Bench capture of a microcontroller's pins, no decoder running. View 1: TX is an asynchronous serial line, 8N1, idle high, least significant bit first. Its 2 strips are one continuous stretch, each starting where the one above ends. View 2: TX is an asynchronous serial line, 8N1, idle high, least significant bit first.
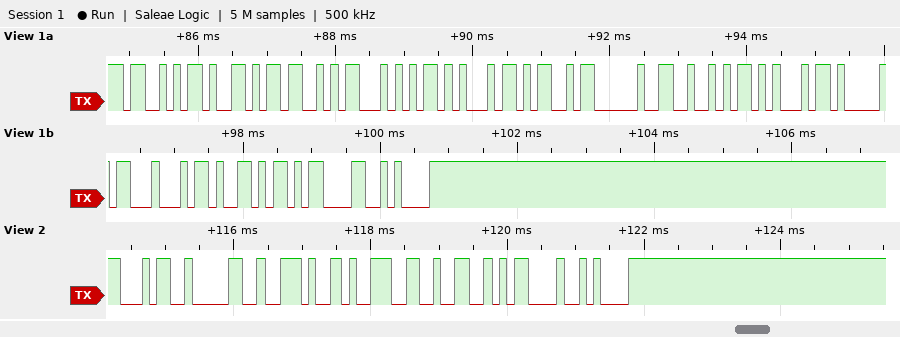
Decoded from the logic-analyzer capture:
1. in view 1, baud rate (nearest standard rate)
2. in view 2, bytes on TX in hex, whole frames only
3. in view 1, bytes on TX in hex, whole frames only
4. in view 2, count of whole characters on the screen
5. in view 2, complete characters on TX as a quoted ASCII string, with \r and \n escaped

9600 baud
34 30 2E 39 32 0D 0A
53 59 53 54 45 4D 20 52 45 41 44 59 0D 0A
7
"40.92\r\n"
